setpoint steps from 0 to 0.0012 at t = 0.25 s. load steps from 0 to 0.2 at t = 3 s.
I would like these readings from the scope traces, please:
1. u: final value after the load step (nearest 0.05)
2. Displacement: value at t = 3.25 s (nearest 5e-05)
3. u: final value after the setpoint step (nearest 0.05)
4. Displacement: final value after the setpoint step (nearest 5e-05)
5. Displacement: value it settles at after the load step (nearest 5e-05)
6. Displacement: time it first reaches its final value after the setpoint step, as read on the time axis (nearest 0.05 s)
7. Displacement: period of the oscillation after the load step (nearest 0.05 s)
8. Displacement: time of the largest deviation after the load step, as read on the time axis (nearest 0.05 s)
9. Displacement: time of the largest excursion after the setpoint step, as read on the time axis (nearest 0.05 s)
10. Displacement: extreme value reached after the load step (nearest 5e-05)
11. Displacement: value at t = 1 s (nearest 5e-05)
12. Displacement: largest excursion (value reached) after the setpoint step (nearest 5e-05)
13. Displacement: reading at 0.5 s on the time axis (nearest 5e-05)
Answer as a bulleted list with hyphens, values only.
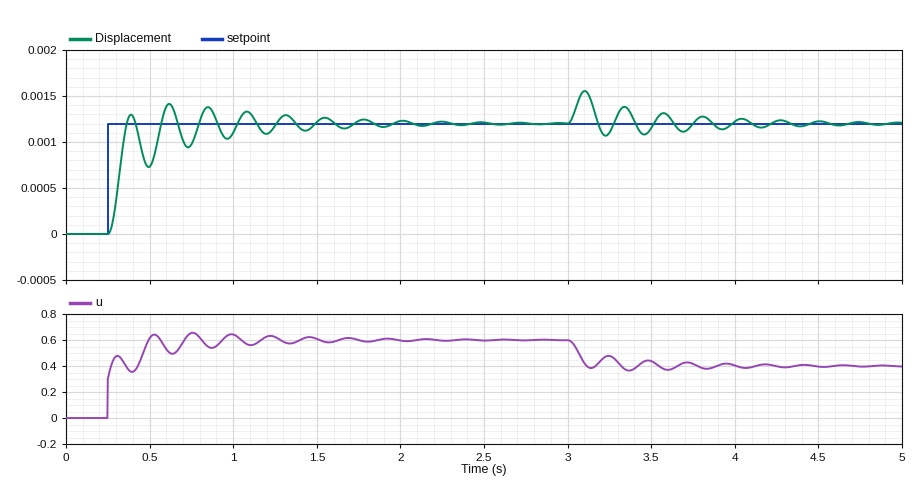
- 0.40
- 0.00110
- 0.60
- 0.00120
- 0.00120
- 0.35 s
- 0.25 s
- 3.10 s
- 0.60 s
- 0.00155
- 0.00110
- 0.00140
- 0.00075
